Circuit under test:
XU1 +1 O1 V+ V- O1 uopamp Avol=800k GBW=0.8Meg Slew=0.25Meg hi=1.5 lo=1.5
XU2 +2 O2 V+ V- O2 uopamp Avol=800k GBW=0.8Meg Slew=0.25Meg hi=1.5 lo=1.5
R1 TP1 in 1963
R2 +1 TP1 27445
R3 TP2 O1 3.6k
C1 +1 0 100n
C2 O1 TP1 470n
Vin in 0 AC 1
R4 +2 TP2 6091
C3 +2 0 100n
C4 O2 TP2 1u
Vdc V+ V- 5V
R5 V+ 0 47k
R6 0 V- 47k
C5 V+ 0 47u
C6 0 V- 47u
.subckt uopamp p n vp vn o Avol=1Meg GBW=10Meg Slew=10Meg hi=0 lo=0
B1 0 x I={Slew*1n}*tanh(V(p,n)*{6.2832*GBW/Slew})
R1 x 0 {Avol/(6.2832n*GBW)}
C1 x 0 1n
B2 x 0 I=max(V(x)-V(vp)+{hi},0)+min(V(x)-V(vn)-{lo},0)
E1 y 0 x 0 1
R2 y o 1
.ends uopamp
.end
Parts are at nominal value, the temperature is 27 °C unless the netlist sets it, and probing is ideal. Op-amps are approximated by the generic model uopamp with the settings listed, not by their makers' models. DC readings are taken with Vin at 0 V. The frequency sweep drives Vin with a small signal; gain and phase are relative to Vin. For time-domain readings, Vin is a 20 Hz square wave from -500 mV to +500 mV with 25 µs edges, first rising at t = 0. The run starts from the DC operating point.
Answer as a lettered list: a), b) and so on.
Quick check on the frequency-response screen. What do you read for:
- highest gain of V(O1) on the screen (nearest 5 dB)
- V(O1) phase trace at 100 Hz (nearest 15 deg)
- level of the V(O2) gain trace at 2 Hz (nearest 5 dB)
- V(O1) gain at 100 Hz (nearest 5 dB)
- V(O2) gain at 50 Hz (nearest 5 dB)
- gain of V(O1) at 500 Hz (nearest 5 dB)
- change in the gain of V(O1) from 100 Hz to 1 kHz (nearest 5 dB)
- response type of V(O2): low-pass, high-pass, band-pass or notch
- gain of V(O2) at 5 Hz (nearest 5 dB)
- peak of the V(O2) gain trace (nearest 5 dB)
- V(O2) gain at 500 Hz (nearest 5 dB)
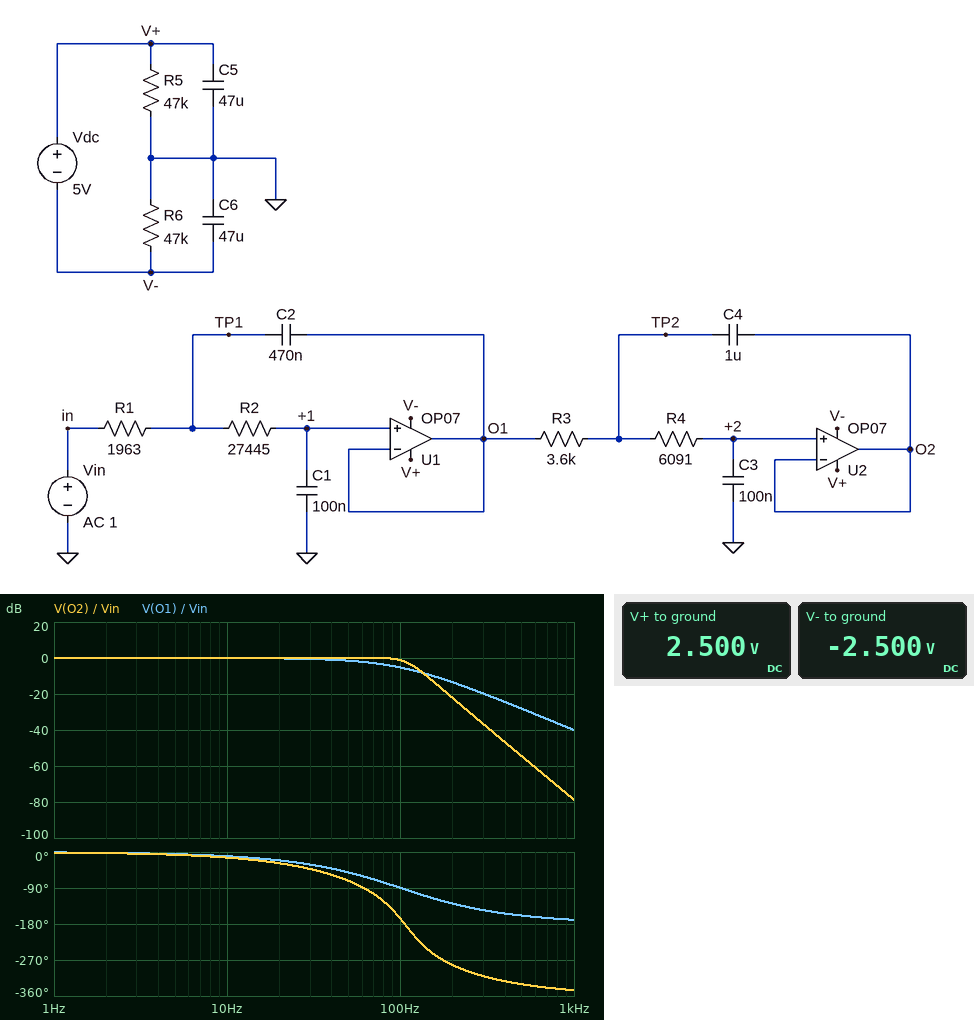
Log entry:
a) 0 dB
b) -90 deg
c) 0 dB
d) -5 dB
e) 0 dB
f) -30 dB
g) -35 dB
h) low-pass
i) 0 dB
j) 0 dB
k) -55 dB
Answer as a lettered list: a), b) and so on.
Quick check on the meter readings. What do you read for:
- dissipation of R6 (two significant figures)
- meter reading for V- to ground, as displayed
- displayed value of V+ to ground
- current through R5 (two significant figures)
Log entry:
a) 130 µW
b) -2.500 V
c) 2.500 V
d) 53 µA
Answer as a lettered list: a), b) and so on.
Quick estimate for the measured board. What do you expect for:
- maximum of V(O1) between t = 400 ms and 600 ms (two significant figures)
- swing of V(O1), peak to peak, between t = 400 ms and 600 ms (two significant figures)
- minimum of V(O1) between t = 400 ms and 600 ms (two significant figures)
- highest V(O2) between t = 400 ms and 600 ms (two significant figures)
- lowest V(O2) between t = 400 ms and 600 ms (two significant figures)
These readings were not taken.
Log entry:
a) 500 mV
b) 1.0 V
c) -500 mV
d) 620 mV
e) -620 mV
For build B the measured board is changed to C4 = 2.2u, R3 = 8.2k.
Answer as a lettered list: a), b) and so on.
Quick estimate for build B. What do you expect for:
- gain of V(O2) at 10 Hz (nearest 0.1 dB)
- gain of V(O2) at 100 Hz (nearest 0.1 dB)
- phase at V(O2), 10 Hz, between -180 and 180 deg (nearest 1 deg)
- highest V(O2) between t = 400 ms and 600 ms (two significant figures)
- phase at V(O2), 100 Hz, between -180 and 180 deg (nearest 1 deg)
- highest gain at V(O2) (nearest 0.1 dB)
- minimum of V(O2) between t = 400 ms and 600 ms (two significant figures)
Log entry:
a) 0.3 dB
b) -16.1 dB
c) -16 deg
d) 870 mV
e) 105 deg
f) 6.3 dB
g) -870 mV
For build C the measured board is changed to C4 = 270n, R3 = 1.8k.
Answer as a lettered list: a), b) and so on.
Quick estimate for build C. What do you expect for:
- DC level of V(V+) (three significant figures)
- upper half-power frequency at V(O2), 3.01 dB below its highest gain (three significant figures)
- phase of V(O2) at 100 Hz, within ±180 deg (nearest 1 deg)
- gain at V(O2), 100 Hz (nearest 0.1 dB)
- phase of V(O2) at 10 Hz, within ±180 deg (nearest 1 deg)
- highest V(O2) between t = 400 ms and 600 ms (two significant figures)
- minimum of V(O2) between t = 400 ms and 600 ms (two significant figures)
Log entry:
a) 2.50 V
b) 71.4 Hz
c) -119 deg
d) -5.4 dB
e) -13 deg
f) 500 mV
g) -500 mV
